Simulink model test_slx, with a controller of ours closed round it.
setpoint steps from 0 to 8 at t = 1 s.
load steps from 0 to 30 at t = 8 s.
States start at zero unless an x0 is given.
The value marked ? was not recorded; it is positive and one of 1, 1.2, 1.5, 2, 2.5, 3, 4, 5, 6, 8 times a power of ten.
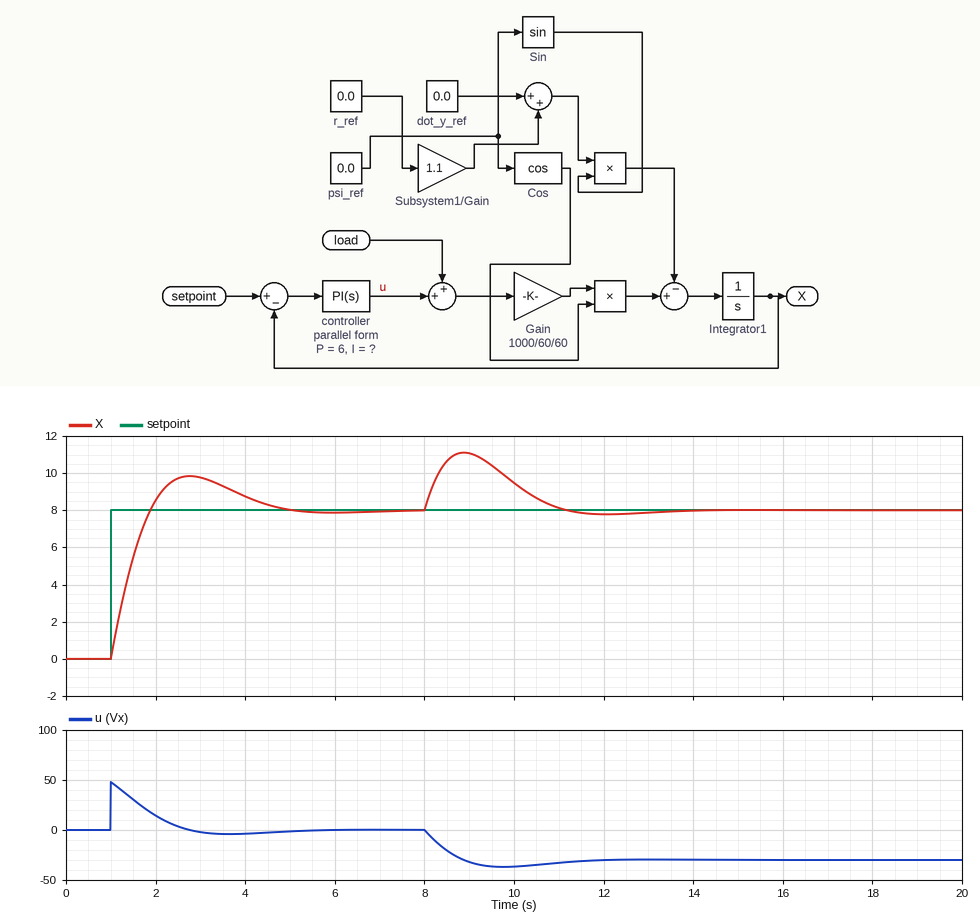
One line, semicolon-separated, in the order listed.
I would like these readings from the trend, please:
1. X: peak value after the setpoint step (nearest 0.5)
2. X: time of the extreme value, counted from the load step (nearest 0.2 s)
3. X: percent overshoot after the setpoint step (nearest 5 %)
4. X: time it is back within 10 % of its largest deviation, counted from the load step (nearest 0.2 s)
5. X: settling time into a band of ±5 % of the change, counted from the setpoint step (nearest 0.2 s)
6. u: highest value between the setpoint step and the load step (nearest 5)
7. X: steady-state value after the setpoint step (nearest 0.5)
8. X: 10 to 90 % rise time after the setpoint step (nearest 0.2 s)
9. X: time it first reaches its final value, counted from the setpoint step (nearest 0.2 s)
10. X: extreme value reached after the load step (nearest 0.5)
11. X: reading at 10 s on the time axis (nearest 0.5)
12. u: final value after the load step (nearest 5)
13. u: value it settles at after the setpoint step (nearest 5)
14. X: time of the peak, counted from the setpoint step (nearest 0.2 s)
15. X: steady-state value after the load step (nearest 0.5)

10.0; 0.8 s; 25 %; 2.8 s; 3.4 s; 50; 8.0; 0.6 s; 0.8 s; 11.0; 9.5; -30; 0; 1.8 s; 8.0
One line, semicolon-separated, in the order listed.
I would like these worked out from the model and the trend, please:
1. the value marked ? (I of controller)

6
